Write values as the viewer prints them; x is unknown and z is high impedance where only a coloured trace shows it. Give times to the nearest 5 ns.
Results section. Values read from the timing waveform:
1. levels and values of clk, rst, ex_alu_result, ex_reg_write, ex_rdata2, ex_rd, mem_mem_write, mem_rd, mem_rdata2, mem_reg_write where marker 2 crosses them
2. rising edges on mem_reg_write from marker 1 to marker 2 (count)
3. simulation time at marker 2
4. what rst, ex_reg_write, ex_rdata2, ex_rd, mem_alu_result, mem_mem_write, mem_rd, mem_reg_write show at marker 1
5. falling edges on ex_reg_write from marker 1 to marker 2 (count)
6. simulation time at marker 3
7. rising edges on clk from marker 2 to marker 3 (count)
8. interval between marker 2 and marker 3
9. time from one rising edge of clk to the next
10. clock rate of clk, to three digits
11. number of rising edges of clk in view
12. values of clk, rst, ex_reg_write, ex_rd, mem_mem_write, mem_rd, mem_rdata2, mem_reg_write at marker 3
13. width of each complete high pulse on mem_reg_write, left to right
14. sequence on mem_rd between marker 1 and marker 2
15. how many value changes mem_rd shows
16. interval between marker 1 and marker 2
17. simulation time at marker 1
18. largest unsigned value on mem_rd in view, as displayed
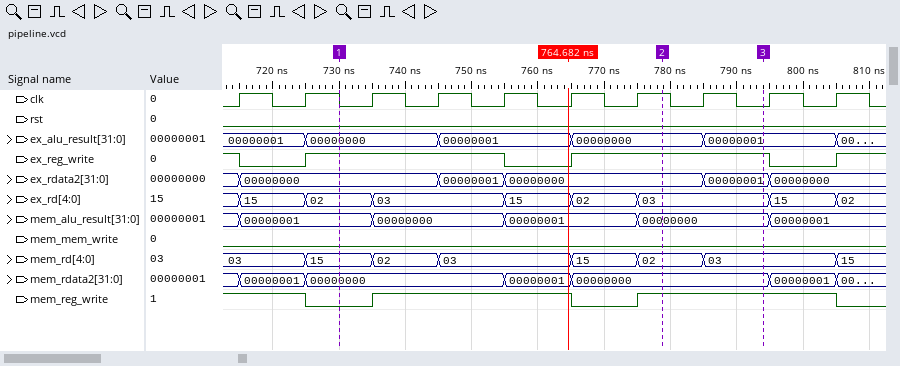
clk=1, rst=0, ex_alu_result=00000000, ex_reg_write=1, ex_rdata2=00000000, ex_rd=03, mem_mem_write=0, mem_rd=02, mem_rdata2=00000000, mem_reg_write=1
2
780 ns
rst=0, ex_reg_write=1, ex_rdata2=00000000, ex_rd=02, mem_alu_result=00000001, mem_mem_write=0, mem_rd=15, mem_reg_write=0
1
795 ns
1
15 ns
10 ns
100 MHz
10
clk=0, rst=0, ex_reg_write=1, ex_rd=03, mem_mem_write=0, mem_rd=03, mem_rdata2=00000000, mem_reg_write=1
30 ns, 30 ns
15, 02, 03, 15, 02
7
50 ns
730 ns
15
